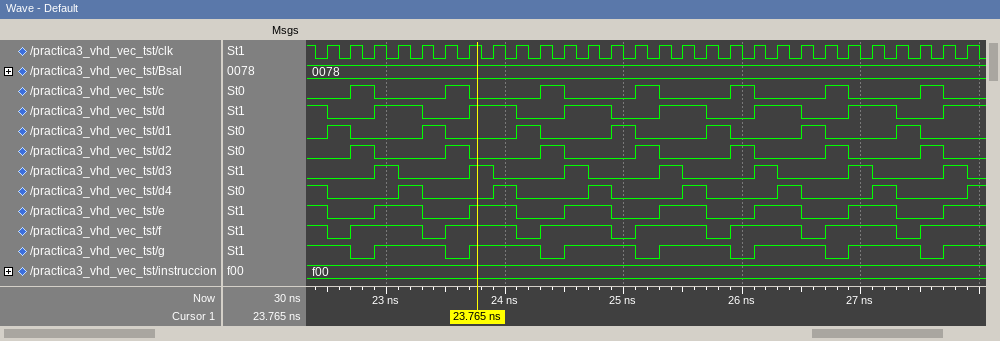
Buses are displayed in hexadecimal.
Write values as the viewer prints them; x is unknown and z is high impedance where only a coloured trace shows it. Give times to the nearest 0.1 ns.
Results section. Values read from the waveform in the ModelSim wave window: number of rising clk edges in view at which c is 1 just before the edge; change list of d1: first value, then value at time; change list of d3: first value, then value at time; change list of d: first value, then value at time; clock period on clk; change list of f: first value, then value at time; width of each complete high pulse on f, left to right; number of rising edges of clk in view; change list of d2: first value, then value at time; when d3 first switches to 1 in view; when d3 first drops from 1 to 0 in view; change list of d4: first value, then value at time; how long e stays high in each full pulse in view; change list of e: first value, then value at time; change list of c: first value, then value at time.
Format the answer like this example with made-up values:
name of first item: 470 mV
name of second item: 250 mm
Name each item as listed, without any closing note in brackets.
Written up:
number of rising clk edges in view at which c is 1 just before the edge: 7
change list of d1: first value, then value at time: 0, 1 at 22.5 ns, 0 at 22.7 ns, 1 at 23.3 ns, 0 at 23.5 ns, 1 at 24.1 ns, 0 at 24.3 ns, 1 at 24.9 ns, 0 at 25.1 ns, 1 at 25.7 ns, 0 at 25.9 ns, 1 at 26.5 ns, 0 at 26.7 ns, 1 at 27.3 ns, 0 at 27.5 ns
change list of d3: first value, then value at time: 0, 1 at 22.9 ns, 0 at 23.1 ns, 1 at 23.7 ns, 0 at 23.9 ns, 1 at 24.5 ns, 0 at 24.7 ns, 1 at 25.3 ns, 0 at 25.5 ns, 1 at 26.1 ns, 0 at 26.3 ns, 1 at 26.9 ns, 0 at 27.1 ns, 1 at 27.7 ns, 0 at 27.9 ns
change list of d: first value, then value at time: 1, 0 at 22.5 ns, 1 at 22.9 ns, 0 at 23.3 ns, 1 at 23.7 ns, 0 at 24.1 ns, 1 at 24.5 ns, 0 at 24.9 ns, 1 at 25.3 ns, 0 at 25.7 ns, 1 at 26.1 ns, 0 at 26.5 ns, 1 at 26.9 ns, 0 at 27.3 ns, 1 at 27.7 ns
clock period on clk: 0.2 ns
change list of f: first value, then value at time: 1, 0 at 22.5 ns, 1 at 22.7 ns, 0 at 23.3 ns, 1 at 23.5 ns, 0 at 24.1 ns, 1 at 24.3 ns, 0 at 24.9 ns, 1 at 25.1 ns, 0 at 25.7 ns, 1 at 25.9 ns, 0 at 26.5 ns, 1 at 26.7 ns, 0 at 27.3 ns, 1 at 27.5 ns
width of each complete high pulse on f, left to right: 0.6 ns, 0.6 ns, 0.6 ns, 0.6 ns, 0.6 ns, 0.6 ns
number of rising edges of clk in view: 28
change list of d2: first value, then value at time: 0, 1 at 22.7 ns, 0 at 22.9 ns, 1 at 23.5 ns, 0 at 23.7 ns, 1 at 24.3 ns, 0 at 24.5 ns, 1 at 25.1 ns, 0 at 25.3 ns, 1 at 25.9 ns, 0 at 26.1 ns, 1 at 26.7 ns, 0 at 26.9 ns, 1 at 27.5 ns, 0 at 27.7 ns
when d3 first switches to 1 in view: 22.9 ns
when d3 first drops from 1 to 0 in view: 23.1 ns
change list of d4: first value, then value at time: 1, 0 at 22.5 ns, 1 at 23.1 ns, 0 at 23.3 ns, 1 at 23.9 ns, 0 at 24.1 ns, 1 at 24.7 ns, 0 at 24.9 ns, 1 at 25.5 ns, 0 at 25.7 ns, 1 at 26.3 ns, 0 at 26.5 ns, 1 at 27.1 ns, 0 at 27.3 ns, 1 at 27.9 ns
how long e stays high in each full pulse in view: 0.4 ns, 0.4 ns, 0.4 ns, 0.4 ns, 0.4 ns, 0.4 ns
change list of e: first value, then value at time: 1, 0 at 22.5 ns, 1 at 22.9 ns, 0 at 23.3 ns, 1 at 23.7 ns, 0 at 24.1 ns, 1 at 24.5 ns, 0 at 24.9 ns, 1 at 25.3 ns, 0 at 25.7 ns, 1 at 26.1 ns, 0 at 26.5 ns, 1 at 26.9 ns, 0 at 27.3 ns, 1 at 27.7 ns
change list of c: first value, then value at time: 0, 1 at 22.7 ns, 0 at 22.9 ns, 1 at 23.5 ns, 0 at 23.7 ns, 1 at 24.3 ns, 0 at 24.5 ns, 1 at 25.1 ns, 0 at 25.3 ns, 1 at 25.9 ns, 0 at 26.1 ns, 1 at 26.7 ns, 0 at 26.9 ns, 1 at 27.5 ns, 0 at 27.7 ns
